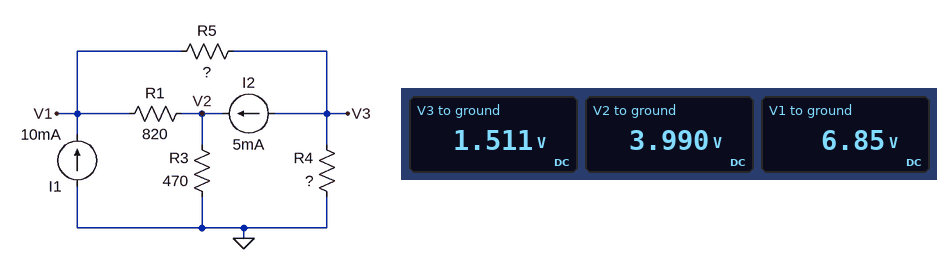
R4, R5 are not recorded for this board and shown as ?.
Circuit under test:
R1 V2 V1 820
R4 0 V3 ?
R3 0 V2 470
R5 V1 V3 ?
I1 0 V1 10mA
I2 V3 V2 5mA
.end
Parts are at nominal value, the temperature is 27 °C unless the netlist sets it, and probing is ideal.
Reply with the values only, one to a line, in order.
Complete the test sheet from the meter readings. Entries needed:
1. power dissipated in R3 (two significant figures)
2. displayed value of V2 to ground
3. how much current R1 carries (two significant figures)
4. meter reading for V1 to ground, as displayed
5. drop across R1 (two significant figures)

34 mW
3.990 V
3.5 mA
6.85 V
2.9 V
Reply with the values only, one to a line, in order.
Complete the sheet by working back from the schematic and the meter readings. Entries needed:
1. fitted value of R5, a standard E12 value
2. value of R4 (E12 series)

820 Ω
1 kΩ
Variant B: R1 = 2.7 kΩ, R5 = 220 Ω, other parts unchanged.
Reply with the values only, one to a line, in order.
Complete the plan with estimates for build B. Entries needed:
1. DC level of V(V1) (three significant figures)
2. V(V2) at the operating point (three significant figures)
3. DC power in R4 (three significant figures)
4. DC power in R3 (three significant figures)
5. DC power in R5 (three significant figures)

5.85 V
2.87 V
15.2 mW
17.5 mW
17.4 mW
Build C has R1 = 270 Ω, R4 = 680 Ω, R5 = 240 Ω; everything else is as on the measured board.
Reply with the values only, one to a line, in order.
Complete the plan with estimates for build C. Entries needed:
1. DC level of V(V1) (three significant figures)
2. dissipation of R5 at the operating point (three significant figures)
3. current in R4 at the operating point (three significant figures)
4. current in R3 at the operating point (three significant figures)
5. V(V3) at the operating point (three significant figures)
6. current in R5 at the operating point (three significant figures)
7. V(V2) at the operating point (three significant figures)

3.89 V
15.1 mW
2.92 mA
7.08 mA
1.99 V
7.92 mA
3.33 V
